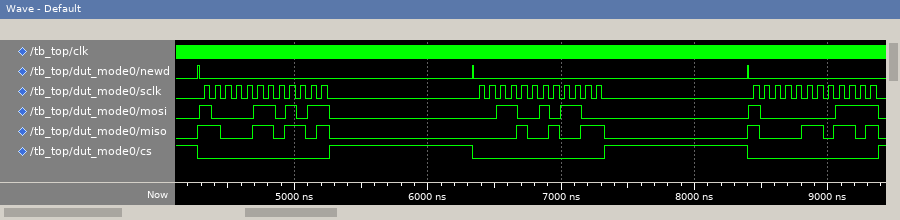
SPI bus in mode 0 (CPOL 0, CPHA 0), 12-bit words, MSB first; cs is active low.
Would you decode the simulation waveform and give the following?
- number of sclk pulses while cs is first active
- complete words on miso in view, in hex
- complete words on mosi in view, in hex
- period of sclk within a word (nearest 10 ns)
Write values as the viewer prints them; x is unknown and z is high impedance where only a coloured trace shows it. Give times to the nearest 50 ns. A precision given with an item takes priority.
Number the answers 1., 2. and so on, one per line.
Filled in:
1. 12
2. C6D, 093, 86D
3. 86B, 32C, 80F
4. 80 ns
